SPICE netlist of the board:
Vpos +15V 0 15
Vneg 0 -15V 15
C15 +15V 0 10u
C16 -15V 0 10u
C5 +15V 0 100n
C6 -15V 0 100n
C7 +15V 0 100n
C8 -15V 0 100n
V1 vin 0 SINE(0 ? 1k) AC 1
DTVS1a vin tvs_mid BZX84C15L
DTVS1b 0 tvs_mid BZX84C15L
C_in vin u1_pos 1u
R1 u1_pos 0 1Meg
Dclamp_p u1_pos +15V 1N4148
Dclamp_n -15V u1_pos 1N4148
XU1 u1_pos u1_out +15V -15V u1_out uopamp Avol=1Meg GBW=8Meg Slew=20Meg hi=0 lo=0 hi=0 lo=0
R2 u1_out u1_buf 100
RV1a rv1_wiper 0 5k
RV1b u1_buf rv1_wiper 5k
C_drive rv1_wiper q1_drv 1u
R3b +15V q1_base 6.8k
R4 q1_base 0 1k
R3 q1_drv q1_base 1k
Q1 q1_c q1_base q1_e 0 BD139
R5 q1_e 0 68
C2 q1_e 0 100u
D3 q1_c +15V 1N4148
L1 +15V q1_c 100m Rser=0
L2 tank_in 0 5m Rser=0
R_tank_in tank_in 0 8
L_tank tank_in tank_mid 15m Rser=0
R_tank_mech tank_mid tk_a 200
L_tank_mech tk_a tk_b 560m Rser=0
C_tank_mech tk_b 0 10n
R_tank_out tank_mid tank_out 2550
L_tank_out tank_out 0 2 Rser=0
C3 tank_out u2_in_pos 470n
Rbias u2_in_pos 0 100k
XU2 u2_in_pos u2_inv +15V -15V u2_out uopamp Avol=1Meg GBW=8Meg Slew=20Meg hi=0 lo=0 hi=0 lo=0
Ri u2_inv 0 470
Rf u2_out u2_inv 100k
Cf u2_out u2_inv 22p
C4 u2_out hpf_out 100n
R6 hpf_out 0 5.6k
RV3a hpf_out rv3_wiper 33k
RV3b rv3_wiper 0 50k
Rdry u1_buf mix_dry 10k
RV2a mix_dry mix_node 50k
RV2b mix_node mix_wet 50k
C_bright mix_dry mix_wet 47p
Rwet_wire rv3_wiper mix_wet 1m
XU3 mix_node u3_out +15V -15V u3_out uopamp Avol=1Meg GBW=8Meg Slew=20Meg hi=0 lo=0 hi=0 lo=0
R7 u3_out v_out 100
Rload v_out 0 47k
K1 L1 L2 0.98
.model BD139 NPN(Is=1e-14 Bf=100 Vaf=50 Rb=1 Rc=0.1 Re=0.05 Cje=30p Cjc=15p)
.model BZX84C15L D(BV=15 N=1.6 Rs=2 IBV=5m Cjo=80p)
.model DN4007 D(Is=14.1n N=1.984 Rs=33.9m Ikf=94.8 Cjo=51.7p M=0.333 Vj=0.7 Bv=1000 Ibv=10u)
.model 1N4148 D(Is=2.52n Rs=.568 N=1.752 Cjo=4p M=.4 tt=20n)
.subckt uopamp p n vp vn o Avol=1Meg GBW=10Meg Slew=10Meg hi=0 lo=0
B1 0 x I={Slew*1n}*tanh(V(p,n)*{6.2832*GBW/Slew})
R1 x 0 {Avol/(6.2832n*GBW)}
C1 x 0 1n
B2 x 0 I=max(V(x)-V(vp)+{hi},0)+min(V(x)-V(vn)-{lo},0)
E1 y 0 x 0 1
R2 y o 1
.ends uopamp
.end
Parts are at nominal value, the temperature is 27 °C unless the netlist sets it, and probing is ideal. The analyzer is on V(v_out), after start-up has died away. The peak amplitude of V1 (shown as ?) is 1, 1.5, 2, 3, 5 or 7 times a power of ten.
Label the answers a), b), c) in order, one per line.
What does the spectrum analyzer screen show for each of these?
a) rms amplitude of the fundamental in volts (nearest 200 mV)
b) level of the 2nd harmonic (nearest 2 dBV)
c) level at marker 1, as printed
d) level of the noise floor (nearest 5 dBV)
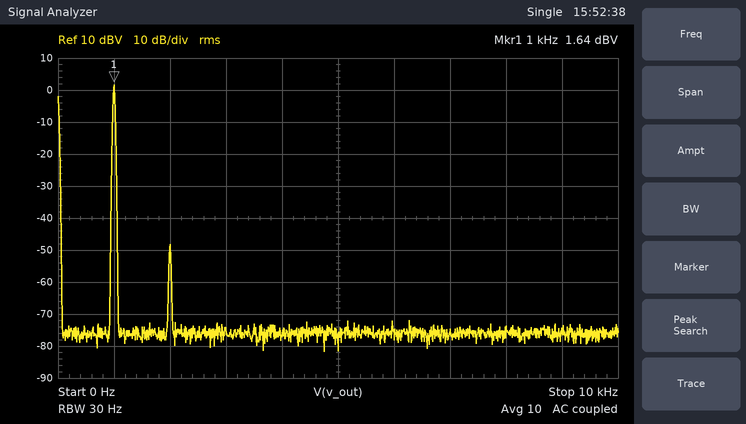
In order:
a) 1.2 V
b) -48 dBV
c) 1.64 dBV
d) -75 dBV
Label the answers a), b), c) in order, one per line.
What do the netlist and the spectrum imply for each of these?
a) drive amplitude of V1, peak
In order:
a) 70 mV
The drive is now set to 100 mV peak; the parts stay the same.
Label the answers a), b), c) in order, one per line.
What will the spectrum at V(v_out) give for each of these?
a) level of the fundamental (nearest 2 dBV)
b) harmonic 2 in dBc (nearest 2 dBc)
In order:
a) 4 dBV
b) -46 dBc
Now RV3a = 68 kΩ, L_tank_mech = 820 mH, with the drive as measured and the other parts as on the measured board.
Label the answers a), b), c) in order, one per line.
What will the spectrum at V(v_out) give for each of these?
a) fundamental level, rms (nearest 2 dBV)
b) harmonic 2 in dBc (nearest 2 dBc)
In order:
a) -2 dBV
b) -52 dBc
